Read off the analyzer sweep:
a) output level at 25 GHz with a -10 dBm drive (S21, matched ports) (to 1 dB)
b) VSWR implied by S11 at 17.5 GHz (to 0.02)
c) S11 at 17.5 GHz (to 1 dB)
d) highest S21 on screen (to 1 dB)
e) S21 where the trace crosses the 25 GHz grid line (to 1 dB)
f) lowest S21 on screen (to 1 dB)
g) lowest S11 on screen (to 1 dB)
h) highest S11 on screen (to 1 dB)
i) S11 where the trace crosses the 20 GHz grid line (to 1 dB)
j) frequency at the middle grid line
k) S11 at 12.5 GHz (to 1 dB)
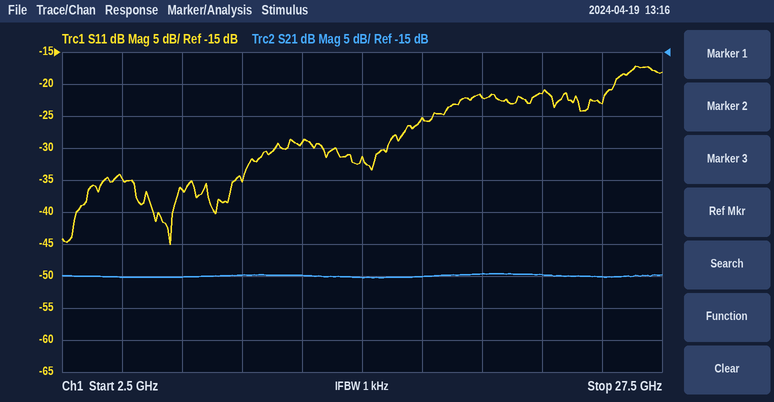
-60 dBm
1.12
-25 dB
-50 dB
-50 dB
-50 dB
-45 dB
-17 dB
-22 dB
15 GHz
-29 dB
